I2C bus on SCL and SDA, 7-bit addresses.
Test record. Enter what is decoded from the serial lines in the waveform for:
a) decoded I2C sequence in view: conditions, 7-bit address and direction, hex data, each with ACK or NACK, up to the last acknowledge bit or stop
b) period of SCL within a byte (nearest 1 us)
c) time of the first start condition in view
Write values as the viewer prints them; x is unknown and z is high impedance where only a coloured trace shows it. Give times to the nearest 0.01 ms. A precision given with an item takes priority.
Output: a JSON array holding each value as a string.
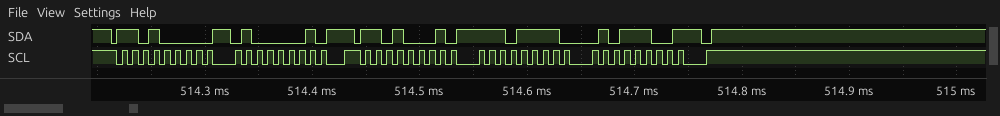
["start, address 68 write ACK, 41 ACK, repeated start, address 68 read ACK, EF ACK, 5C NACK, stop", "10 us", "514.21 ms"]
